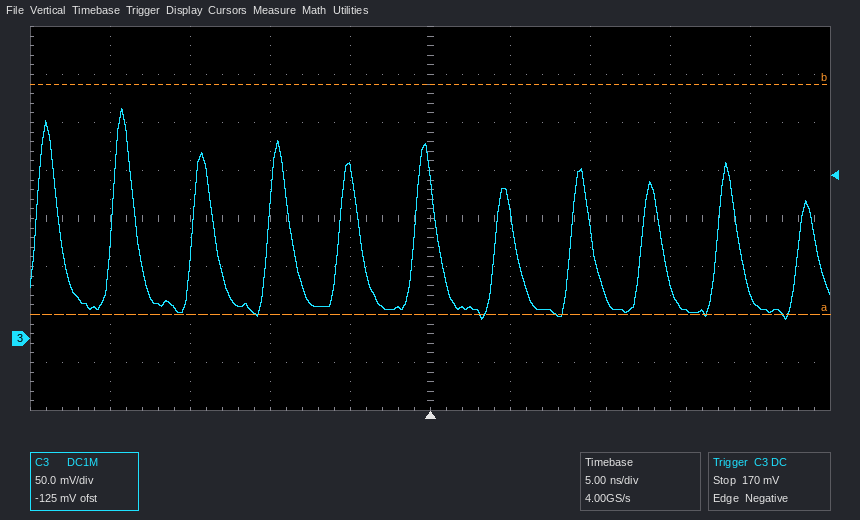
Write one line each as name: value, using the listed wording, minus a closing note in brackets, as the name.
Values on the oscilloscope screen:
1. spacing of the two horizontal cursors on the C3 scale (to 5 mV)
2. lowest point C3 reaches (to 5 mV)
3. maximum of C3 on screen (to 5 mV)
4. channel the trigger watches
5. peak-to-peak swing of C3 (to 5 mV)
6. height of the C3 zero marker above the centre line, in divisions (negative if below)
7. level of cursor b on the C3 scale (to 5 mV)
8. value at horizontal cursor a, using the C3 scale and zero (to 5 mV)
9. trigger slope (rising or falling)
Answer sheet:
spacing of the two horizontal cursors on the C3 scale: 240 mV
lowest point C3 reaches: 20 mV
maximum of C3 on screen: 240 mV
channel the trigger watches: C3
peak-to-peak swing of C3: 220 mV
height of the C3 zero marker above the centre line, in divisions: -2.5 div
level of cursor b on the C3 scale: 265 mV
value at horizontal cursor a, using the C3 scale and zero: 25 mV
trigger slope: falling
